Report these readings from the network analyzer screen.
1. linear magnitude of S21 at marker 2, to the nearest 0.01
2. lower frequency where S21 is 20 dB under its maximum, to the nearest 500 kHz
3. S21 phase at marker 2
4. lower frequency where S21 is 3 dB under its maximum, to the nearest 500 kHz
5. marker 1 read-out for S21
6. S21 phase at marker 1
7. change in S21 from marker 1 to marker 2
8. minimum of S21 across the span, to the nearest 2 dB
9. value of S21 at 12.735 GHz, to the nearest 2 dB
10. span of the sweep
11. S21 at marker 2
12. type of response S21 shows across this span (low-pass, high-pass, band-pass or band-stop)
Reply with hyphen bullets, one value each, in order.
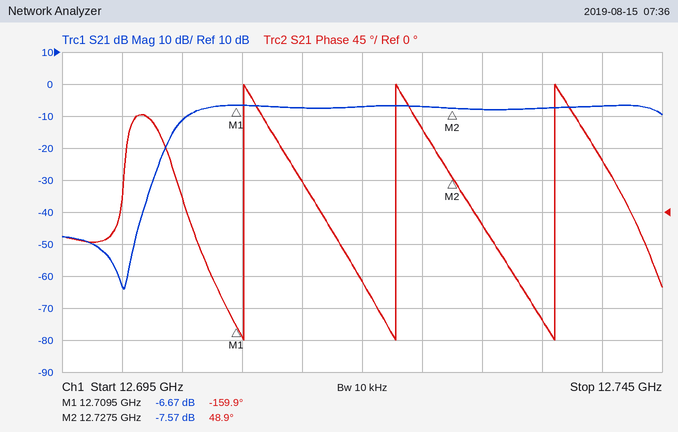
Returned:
- 0.42
- 12.7030 GHz
- 48.9°
- 12.7055 GHz
- -6.67 dB
- -159.9°
- -0.90 dB
- -64 dB
- -8 dB
- 50 MHz
- -7.57 dB
- high-pass
